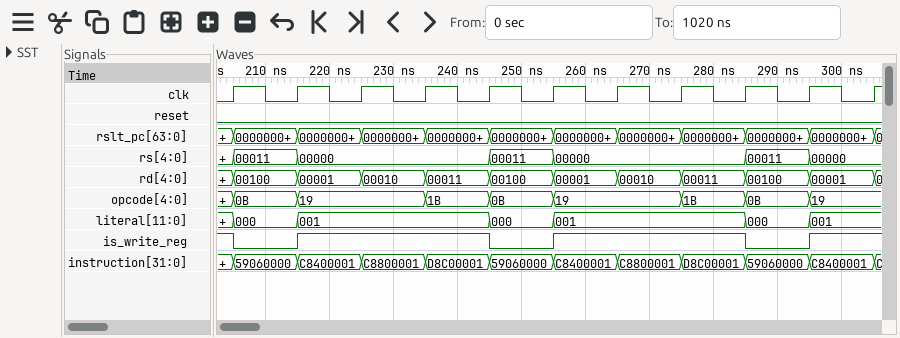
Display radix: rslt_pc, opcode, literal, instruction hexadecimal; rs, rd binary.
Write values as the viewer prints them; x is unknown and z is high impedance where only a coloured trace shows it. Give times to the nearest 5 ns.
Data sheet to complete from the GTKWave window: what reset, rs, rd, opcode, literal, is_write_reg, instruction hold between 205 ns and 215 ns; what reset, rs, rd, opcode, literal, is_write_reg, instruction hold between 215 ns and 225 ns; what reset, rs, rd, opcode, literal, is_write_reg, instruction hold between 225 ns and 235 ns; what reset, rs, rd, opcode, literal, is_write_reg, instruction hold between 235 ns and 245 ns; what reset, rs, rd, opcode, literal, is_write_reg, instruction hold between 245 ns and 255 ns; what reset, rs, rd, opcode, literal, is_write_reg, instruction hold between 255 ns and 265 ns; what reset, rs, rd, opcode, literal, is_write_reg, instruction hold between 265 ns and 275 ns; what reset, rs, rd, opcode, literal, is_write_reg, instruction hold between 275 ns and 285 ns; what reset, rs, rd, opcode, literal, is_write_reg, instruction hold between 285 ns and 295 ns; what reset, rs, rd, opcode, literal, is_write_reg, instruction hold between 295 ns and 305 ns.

reset=0, rs=00011, rd=00100, opcode=0B, literal=000, is_write_reg=0, instruction=59060000
reset=0, rs=00000, rd=00001, opcode=19, literal=001, is_write_reg=1, instruction=C8400001
reset=0, rs=00000, rd=00010, opcode=19, literal=001, is_write_reg=1, instruction=C8800001
reset=0, rs=00000, rd=00011, opcode=1B, literal=001, is_write_reg=1, instruction=D8C00001
reset=0, rs=00011, rd=00100, opcode=0B, literal=000, is_write_reg=0, instruction=59060000
reset=0, rs=00000, rd=00001, opcode=19, literal=001, is_write_reg=1, instruction=C8400001
reset=0, rs=00000, rd=00010, opcode=19, literal=001, is_write_reg=1, instruction=C8800001
reset=0, rs=00000, rd=00011, opcode=1B, literal=001, is_write_reg=1, instruction=D8C00001
reset=0, rs=00011, rd=00100, opcode=0B, literal=000, is_write_reg=0, instruction=59060000
reset=0, rs=00000, rd=00001, opcode=19, literal=001, is_write_reg=1, instruction=C8400001
